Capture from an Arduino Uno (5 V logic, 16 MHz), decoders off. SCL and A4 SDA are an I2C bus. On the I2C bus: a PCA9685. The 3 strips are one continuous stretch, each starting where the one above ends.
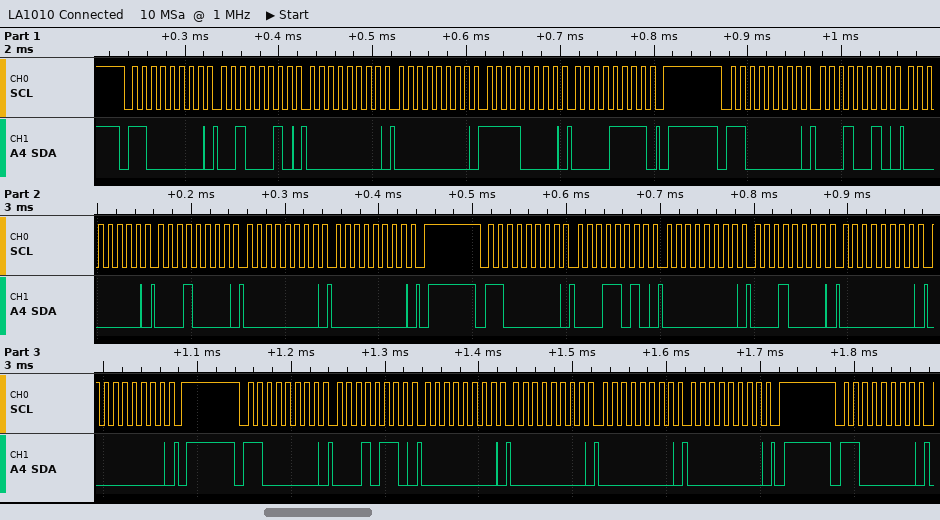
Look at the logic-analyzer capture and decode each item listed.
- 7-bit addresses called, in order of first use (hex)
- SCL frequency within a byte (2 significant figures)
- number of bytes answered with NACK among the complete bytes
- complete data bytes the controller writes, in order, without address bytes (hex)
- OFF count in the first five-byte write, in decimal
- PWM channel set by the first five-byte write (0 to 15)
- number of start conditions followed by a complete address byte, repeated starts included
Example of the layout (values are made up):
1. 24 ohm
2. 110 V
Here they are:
1. 0x60
2. 100 kHz
3. 0
4. 22 00 00 F0 0F 12 00 10 00 00 1A 00 10 00 00 16 00 00 00 00
5. 4080
6. 7
7. 5
